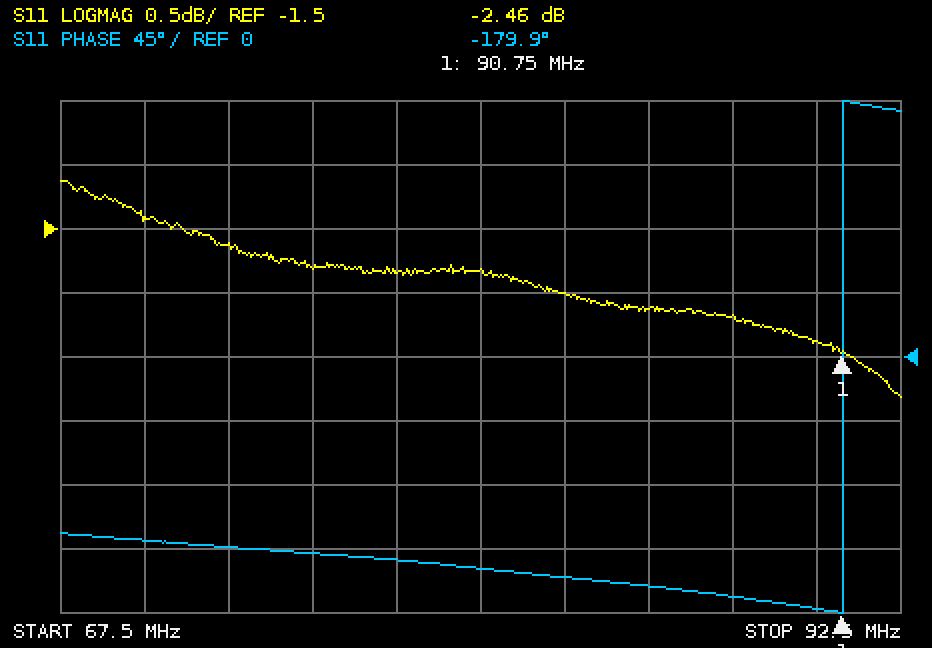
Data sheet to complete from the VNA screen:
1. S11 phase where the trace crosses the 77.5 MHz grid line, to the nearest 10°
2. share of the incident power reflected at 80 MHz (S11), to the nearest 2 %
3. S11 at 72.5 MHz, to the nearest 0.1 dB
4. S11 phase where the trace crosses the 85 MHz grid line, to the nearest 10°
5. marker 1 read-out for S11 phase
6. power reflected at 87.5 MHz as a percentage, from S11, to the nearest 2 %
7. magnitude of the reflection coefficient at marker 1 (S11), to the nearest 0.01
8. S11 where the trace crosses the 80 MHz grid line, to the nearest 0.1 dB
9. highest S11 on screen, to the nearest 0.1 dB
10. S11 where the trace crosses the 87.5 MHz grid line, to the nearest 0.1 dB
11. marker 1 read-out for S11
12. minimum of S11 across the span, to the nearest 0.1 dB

-140°
66 %
-1.6 dB
-160°
-179.9°
60 %
0.75
-1.8 dB
-1.1 dB
-2.2 dB
-2.46 dB
-2.8 dB
